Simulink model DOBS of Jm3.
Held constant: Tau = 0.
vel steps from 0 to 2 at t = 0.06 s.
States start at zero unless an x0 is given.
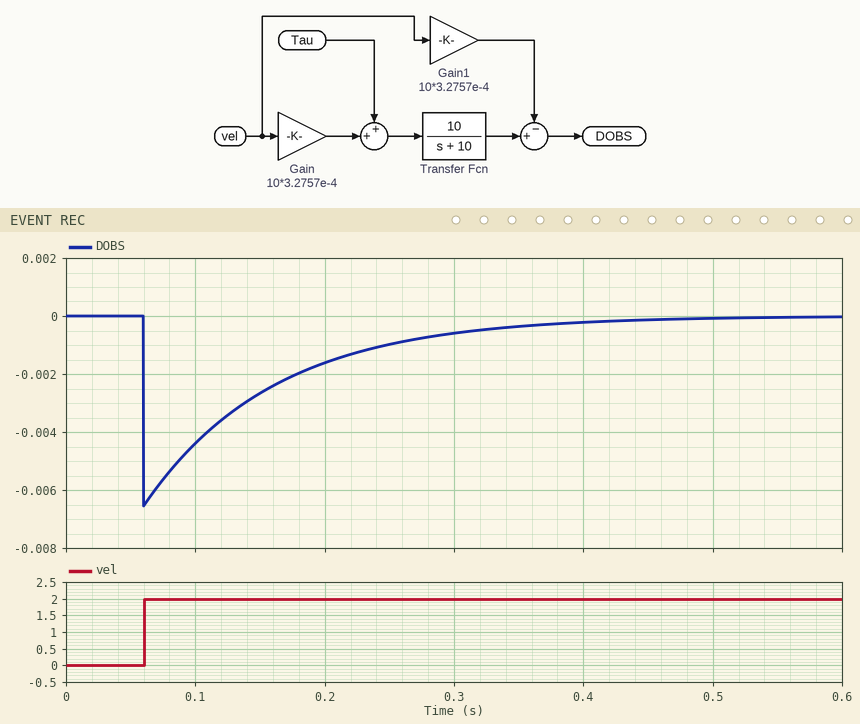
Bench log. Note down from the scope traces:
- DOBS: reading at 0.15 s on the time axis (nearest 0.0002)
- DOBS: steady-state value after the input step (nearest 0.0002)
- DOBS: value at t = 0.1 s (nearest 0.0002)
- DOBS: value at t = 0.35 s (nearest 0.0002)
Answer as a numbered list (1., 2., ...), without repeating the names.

1. -0.0026
2. 0.0000
3. -0.0044
4. -0.0004
